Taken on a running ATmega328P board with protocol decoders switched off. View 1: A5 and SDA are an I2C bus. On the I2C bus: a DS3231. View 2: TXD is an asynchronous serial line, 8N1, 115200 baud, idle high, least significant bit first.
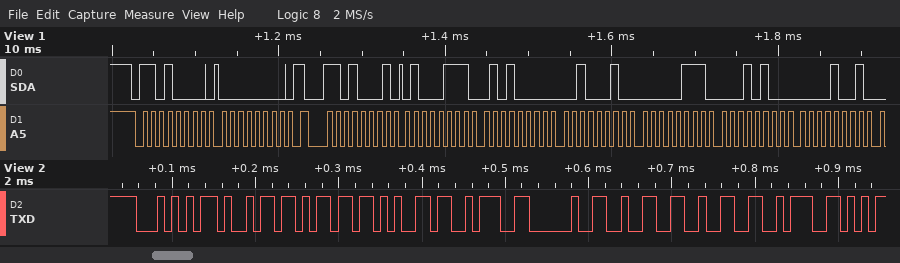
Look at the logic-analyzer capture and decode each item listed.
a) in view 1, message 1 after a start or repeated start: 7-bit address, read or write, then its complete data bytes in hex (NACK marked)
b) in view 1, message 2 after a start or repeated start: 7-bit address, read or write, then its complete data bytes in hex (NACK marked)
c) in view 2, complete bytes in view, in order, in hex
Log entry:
0x68 write: 00
0x68 read: 47 50 22 07 14 09
0x54 0x69 0x6D 0x65 0x3A 0x20 0x32 0x32 0x3A
